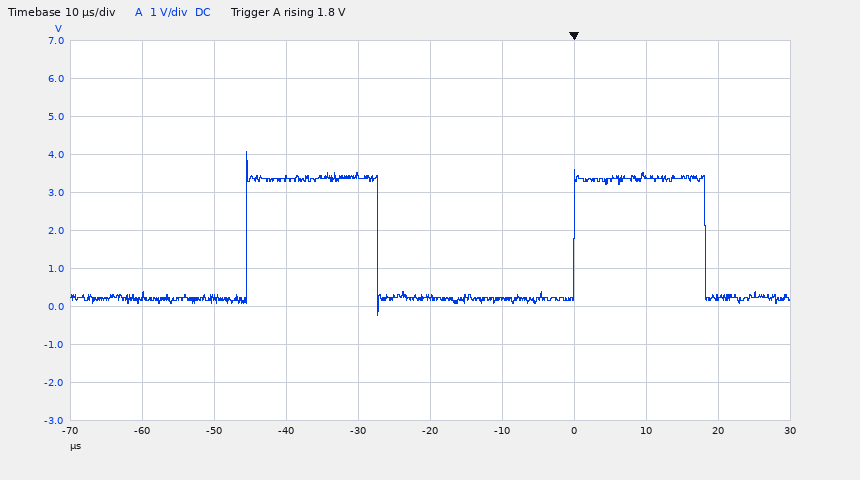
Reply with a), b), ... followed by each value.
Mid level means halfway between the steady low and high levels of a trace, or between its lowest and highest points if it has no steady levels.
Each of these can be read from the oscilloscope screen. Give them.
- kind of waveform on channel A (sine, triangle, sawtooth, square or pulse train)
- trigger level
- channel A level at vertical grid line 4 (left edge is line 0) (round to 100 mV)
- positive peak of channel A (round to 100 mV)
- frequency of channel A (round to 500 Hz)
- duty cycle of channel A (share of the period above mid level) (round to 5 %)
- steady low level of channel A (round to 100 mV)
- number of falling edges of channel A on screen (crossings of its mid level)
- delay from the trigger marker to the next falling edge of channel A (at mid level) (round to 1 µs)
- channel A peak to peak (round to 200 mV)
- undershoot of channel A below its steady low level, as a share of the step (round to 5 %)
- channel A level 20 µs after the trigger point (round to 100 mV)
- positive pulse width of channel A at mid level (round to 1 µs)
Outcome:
a) pulse train
b) 1.8 V
c) 3.4 V
d) 4.1 V
e) 22.0 kHz
f) 40 %
g) 200 mV
h) 2
i) 18 µs
j) 4.4 V
k) 15 %
l) 200 mV
m) 18 µs
